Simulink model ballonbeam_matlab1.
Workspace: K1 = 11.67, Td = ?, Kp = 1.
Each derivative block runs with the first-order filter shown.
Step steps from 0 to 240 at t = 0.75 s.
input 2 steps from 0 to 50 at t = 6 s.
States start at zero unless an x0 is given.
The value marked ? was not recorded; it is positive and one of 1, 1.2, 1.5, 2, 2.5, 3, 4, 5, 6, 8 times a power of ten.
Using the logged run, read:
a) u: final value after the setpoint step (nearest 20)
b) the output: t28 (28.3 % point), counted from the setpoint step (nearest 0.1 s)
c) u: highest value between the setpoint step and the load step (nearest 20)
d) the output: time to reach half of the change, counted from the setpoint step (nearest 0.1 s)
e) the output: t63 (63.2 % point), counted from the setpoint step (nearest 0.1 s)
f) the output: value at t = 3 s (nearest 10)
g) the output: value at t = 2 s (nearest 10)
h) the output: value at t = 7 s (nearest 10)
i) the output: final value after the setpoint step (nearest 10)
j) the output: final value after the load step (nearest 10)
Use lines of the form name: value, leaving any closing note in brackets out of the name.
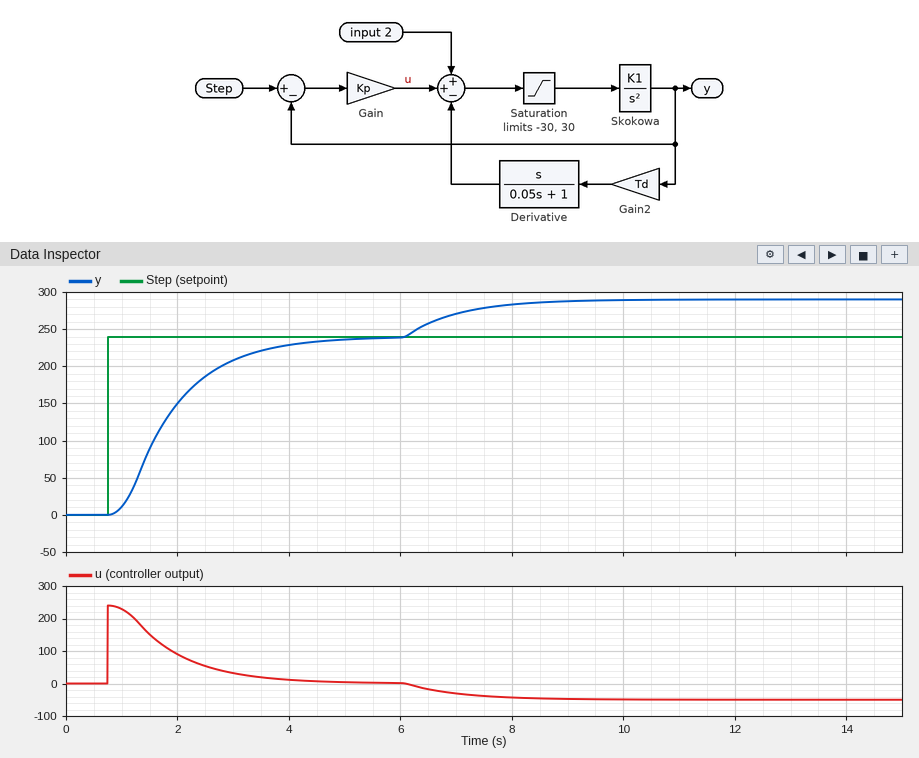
u: final value after the setpoint step: 0
the output: t28 (28.3 % point), counted from the setpoint step: 0.6 s
u: highest value between the setpoint step and the load step: 240
the output: time to reach half of the change, counted from the setpoint step: 1.0 s
the output: t63 (63.2 % point), counted from the setpoint step: 1.3 s
the output: value at t = 3 s: 210
the output: value at t = 2 s: 150
the output: value at t = 7 s: 270
the output: final value after the setpoint step: 240
the output: final value after the load step: 290
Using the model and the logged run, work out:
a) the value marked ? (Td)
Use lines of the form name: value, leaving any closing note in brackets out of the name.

the value marked ?: 1
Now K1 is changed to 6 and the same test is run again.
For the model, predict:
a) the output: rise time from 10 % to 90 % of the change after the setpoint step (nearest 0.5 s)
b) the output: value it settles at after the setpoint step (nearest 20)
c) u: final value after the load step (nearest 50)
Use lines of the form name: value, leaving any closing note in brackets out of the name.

the output: rise time from 10 % to 90 % of the change after the setpoint step: 2.0 s
the output: value it settles at after the setpoint step: 240
u: final value after the load step: -50
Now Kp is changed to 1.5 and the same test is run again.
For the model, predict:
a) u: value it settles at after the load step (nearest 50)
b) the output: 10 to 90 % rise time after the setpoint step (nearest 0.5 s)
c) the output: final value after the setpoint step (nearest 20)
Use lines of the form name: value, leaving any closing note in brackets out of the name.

u: value it settles at after the load step: -50
the output: 10 to 90 % rise time after the setpoint step: 1.5 s
the output: final value after the setpoint step: 240
